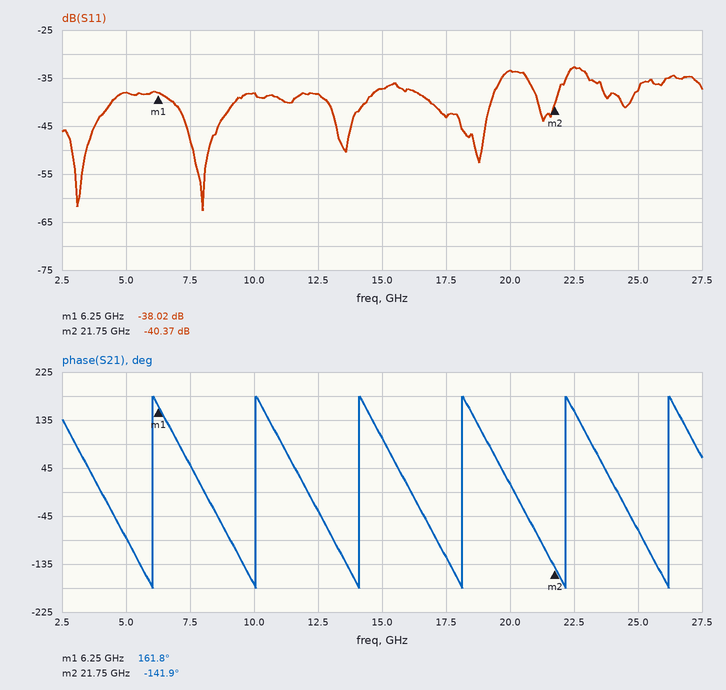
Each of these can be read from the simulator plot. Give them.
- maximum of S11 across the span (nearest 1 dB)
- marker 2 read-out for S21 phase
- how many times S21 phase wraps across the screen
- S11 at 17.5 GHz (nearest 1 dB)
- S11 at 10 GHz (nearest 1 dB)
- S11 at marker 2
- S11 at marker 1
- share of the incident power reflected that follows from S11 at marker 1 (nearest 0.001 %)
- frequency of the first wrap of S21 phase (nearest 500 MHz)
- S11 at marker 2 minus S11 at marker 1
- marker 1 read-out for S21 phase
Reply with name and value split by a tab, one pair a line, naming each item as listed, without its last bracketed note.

maximum of S11 across the span	-33 dB
marker 2 read-out for S21 phase	-141.9°
how many times S21 phase wraps across the screen	6
S11 at 17.5 GHz	-43 dB
S11 at 10 GHz	-38 dB
S11 at marker 2	-40.37 dB
S11 at marker 1	-38.02 dB
share of the incident power reflected that follows from S11 at marker 1	0.016 %
frequency of the first wrap of S21 phase	6.0 GHz
S11 at marker 2 minus S11 at marker 1	-2.35 dB
marker 1 read-out for S21 phase	161.8°
